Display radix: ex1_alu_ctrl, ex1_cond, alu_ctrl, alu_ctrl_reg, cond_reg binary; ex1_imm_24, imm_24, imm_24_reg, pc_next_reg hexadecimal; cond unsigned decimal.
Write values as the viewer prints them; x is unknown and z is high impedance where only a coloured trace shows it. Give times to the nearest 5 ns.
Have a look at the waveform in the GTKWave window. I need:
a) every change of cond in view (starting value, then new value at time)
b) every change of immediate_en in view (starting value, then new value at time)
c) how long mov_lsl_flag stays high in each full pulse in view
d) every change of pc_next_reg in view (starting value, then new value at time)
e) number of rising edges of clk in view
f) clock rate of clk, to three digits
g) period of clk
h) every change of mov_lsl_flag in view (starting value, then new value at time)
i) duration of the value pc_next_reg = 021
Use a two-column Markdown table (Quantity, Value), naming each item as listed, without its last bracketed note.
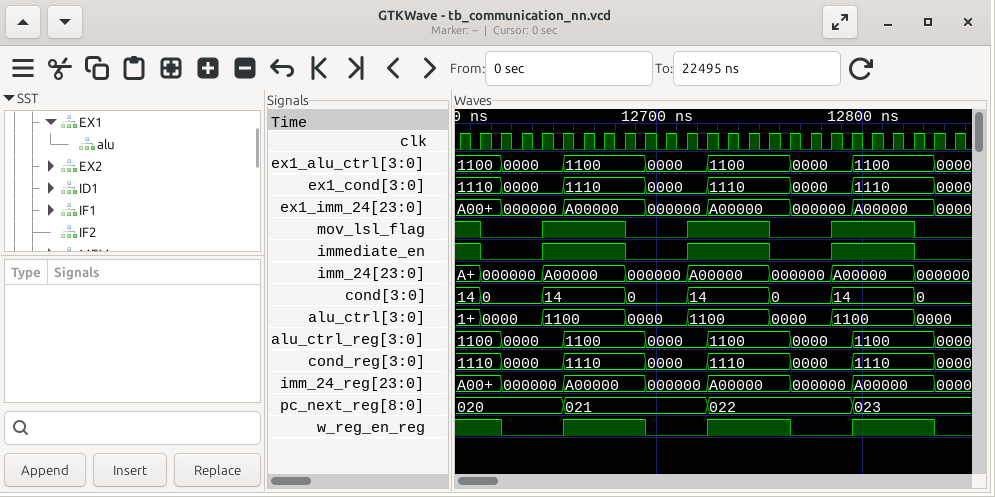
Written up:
| Quantity | Value |
|---|---|
| every change of cond in view | 14, 0 at 12615 ns, 14 at 12645 ns, 0 at 12685 ns, 14 at 12715 ns, 0 at 12755 ns, 14 at 12785 ns, 0 at 12825 ns |
| every change of immediate_en in view | 1, 0 at 12615 ns, 1 at 12645 ns, 0 at 12685 ns, 1 at 12715 ns, 0 at 12755 ns, 1 at 12785 ns, 0 at 12825 ns |
| how long mov_lsl_flag stays high in each full pulse in view | 40 ns, 40 ns, 40 ns |
| every change of pc_next_reg in view | 020, 021 at 12655 ns, 022 at 12725 ns, 023 at 12795 ns |
| number of rising edges of clk in view | 25 |
| clock rate of clk, to three digits | 100 MHz |
| period of clk | 10 ns |
| every change of mov_lsl_flag in view | 1, 0 at 12615 ns, 1 at 12645 ns, 0 at 12685 ns, 1 at 12715 ns, 0 at 12755 ns, 1 at 12785 ns, 0 at 12825 ns |
| duration of the value pc_next_reg = 021 | 70 ns |
